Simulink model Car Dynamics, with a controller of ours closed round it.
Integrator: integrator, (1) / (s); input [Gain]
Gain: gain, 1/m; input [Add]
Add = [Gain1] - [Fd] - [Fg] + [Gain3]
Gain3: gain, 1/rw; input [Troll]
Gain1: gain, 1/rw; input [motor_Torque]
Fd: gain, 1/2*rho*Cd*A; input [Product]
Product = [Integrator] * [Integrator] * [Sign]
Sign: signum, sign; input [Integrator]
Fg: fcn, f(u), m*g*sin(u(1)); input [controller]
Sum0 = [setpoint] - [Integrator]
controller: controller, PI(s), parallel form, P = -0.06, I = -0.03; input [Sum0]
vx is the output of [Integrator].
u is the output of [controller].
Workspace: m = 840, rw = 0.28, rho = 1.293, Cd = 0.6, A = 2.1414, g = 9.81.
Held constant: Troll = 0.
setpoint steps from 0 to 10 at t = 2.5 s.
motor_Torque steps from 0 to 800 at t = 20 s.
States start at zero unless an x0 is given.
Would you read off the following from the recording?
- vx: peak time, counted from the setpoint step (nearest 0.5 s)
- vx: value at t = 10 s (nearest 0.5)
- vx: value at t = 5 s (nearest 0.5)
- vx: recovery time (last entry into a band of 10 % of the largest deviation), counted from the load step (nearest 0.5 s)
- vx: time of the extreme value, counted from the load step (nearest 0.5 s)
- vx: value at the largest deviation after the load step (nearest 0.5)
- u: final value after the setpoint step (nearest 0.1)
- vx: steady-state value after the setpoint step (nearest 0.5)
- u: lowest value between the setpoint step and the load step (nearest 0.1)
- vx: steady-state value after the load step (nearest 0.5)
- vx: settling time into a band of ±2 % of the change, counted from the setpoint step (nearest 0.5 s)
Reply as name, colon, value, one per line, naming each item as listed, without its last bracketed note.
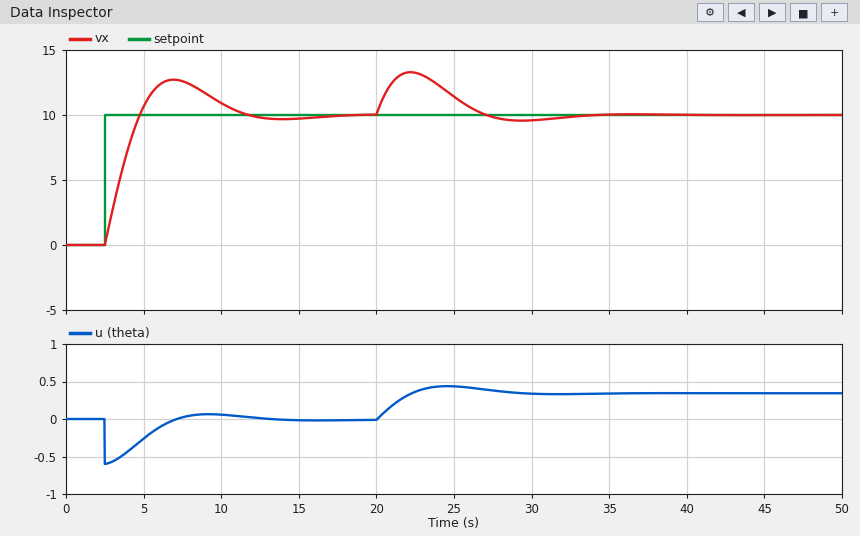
vx: peak time, counted from the setpoint step: 4.5 s
vx: value at t = 10 s: 11.0
vx: value at t = 5 s: 10.5
vx: recovery time (last entry into a band of 10 % of the largest deviation), counted from the load step: 11.0 s
vx: time of the extreme value, counted from the load step: 2.0 s
vx: value at the largest deviation after the load step: 13.5
u: final value after the setpoint step: 0.0
vx: steady-state value after the setpoint step: 10.0
u: lowest value between the setpoint step and the load step: -0.6
vx: steady-state value after the load step: 10.0
vx: settling time into a band of ±2 % of the change, counted from the setpoint step: 13.5 s
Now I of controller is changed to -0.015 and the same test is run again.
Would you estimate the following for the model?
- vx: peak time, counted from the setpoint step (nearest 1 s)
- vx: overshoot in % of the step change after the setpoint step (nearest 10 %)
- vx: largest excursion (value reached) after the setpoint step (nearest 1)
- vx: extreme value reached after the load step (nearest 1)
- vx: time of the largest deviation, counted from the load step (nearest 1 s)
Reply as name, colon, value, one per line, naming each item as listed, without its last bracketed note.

vx: peak time, counted from the setpoint step: 6 s
vx: overshoot in % of the step change after the setpoint step: 20 %
vx: largest excursion (value reached) after the setpoint step: 12
vx: extreme value reached after the load step: 14
vx: time of the largest deviation, counted from the load step: 3 s
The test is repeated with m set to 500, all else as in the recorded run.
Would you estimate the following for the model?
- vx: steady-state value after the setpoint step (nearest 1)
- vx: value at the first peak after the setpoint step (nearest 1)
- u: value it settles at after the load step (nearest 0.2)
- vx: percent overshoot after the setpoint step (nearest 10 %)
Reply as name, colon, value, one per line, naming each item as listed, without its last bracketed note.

vx: steady-state value after the setpoint step: 10
vx: value at the first peak after the setpoint step: 13
u: value it settles at after the load step: 0.6
vx: percent overshoot after the setpoint step: 30 %
